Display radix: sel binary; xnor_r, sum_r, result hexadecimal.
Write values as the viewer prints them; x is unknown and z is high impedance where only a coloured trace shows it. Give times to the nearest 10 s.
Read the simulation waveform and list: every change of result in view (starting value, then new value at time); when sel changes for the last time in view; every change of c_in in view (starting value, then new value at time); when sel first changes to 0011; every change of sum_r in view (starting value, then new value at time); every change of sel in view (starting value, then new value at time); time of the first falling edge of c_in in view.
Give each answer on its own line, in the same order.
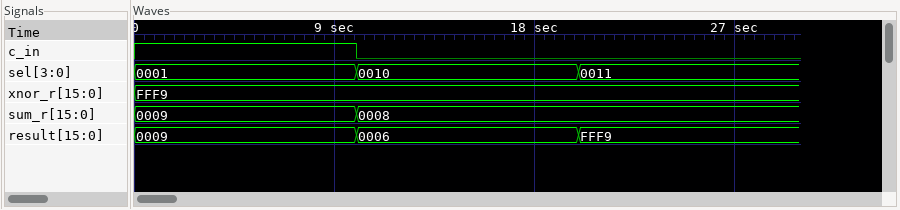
0009, 0006 at 10 s, FFF9 at 20 s
20 s
1, 0 at 10 s
20 s
0009, 0008 at 10 s
0001, 0010 at 10 s, 0011 at 20 s
10 s
